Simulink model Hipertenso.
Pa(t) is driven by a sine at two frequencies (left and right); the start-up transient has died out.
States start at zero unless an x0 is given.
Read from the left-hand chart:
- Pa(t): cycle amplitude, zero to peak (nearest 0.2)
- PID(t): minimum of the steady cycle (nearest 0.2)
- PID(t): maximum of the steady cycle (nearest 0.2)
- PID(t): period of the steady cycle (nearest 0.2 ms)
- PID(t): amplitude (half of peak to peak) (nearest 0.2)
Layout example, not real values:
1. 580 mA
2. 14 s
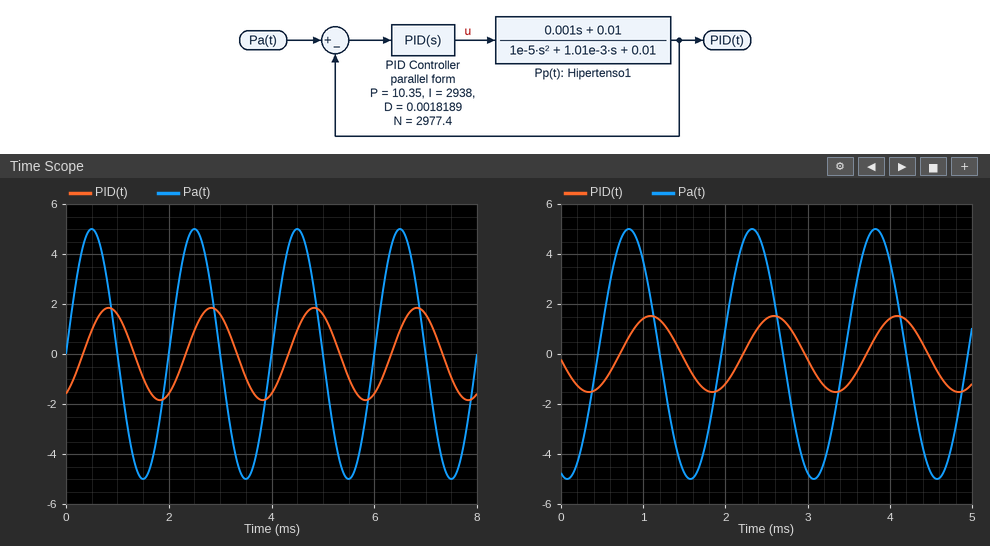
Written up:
1. 5.0
2. -1.8
3. 1.8
4. 2.0 ms
5. 1.8
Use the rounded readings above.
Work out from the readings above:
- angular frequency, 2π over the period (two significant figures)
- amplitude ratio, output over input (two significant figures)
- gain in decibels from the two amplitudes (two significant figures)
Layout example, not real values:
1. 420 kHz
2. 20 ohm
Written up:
1. 3.1 rad/ms
2. 0.36
3. -8.9 dB
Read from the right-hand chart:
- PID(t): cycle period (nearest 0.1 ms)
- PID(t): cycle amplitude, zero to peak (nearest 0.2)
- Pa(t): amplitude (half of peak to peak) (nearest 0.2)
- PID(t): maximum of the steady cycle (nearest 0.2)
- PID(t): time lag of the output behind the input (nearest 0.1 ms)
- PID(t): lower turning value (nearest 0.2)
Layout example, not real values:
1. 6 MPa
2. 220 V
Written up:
1. 1.5 ms
2. 1.6
3. 5.0
4. 1.6
5. 0.3 ms
6. -1.6
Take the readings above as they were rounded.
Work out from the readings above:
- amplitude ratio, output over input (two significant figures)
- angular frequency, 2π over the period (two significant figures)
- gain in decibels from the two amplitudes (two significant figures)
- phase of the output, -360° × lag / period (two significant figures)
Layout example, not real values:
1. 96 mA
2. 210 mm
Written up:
1. 0.32
2. 4.2 rad/ms
3. -9.9 dB
4. -72°
